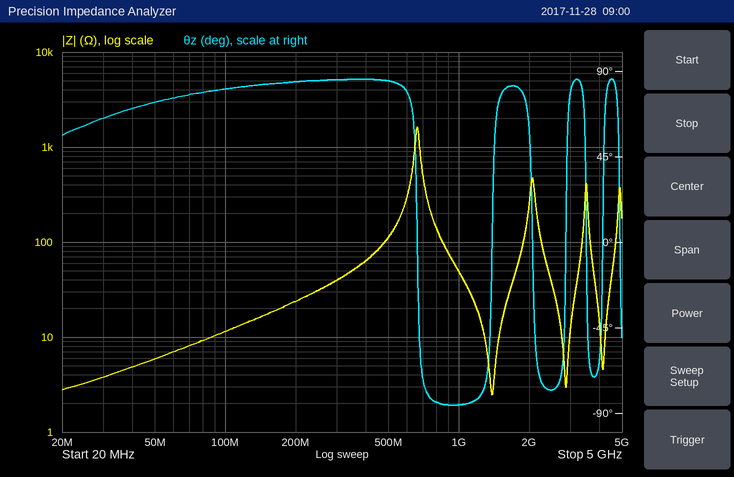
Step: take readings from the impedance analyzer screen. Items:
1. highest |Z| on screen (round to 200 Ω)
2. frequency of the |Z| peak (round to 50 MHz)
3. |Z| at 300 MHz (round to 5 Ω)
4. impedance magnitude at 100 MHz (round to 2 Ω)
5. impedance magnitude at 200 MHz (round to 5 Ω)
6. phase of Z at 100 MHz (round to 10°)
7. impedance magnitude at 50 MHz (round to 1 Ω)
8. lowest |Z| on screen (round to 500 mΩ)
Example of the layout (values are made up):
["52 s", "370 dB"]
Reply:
["1.6 kΩ", "650 MHz", "40 Ω", "12 Ω", "25 Ω", "80°", "6 Ω", "2.5 Ω"]
